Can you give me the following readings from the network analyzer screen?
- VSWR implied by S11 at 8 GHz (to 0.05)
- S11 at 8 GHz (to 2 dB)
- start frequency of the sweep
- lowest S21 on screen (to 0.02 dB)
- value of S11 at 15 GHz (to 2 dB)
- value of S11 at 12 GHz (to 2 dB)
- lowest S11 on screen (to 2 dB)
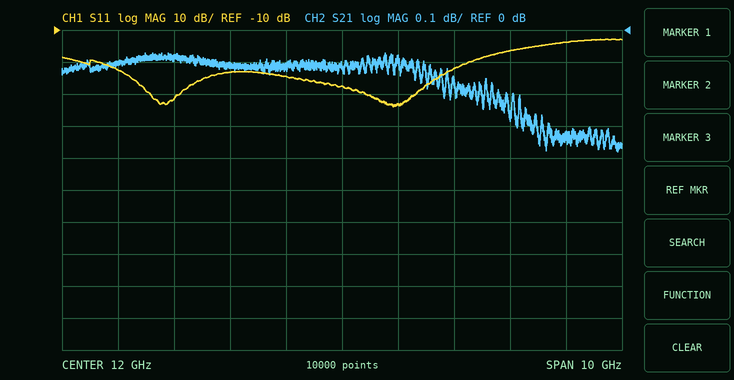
1.15
-22 dB
7 GHz
-0.38 dB
-16 dB
-28 dB
-34 dB
